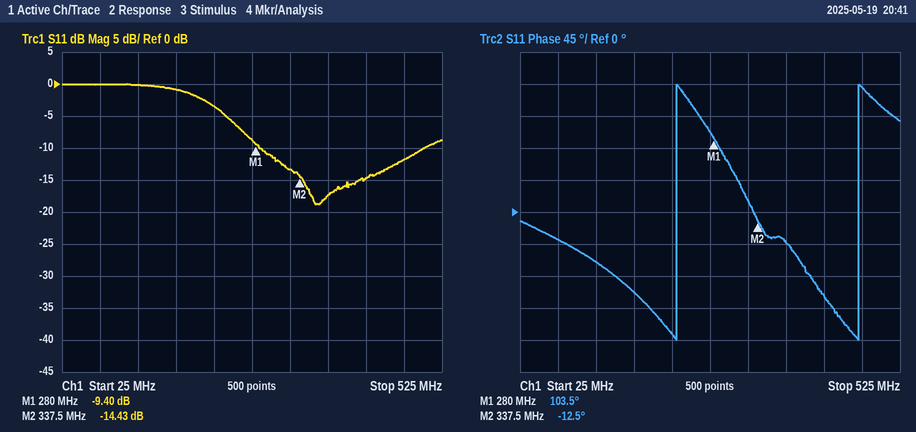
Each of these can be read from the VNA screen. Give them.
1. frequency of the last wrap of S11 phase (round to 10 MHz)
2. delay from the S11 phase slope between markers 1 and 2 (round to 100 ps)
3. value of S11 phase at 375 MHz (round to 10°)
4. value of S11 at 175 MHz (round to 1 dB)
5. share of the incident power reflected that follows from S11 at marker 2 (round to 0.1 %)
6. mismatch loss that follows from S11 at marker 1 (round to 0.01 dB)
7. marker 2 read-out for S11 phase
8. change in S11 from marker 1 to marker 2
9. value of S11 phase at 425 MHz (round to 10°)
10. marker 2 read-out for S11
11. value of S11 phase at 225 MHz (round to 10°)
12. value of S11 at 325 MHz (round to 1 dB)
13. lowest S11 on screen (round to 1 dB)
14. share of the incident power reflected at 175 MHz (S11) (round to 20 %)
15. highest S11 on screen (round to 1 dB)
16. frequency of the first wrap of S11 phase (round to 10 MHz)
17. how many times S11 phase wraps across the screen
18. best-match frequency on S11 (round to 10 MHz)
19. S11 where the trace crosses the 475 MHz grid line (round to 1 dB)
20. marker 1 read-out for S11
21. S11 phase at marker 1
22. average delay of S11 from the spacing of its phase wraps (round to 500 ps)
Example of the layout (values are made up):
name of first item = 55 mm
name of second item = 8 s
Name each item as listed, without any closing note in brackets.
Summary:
frequency of the last wrap of S11 phase = 470 MHz
delay from the S11 phase slope between markers 1 and 2 = 5.6 ns
value of S11 phase at 375 MHz = -40°
value of S11 at 175 MHz = -1 dB
share of the incident power reflected that follows from S11 at marker 2 = 3.6 %
mismatch loss that follows from S11 at marker 1 = 0.53 dB
marker 2 read-out for S11 phase = -12.5°
change in S11 from marker 1 to marker 2 = -5.03 dB
value of S11 phase at 425 MHz = -120°
marker 2 read-out for S11 = -14.43 dB
value of S11 phase at 225 MHz = -170°
value of S11 at 325 MHz = -13 dB
lowest S11 on screen = -19 dB
share of the incident power reflected at 175 MHz (S11) = 80 %
highest S11 on screen = 0 dB
frequency of the first wrap of S11 phase = 230 MHz
how many times S11 phase wraps across the screen = 2
best-match frequency on S11 = 360 MHz
S11 where the trace crosses the 475 MHz grid line = -12 dB
marker 1 read-out for S11 = -9.40 dB
S11 phase at marker 1 = 103.5°
average delay of S11 from the spacing of its phase wraps = 4.0 ns
